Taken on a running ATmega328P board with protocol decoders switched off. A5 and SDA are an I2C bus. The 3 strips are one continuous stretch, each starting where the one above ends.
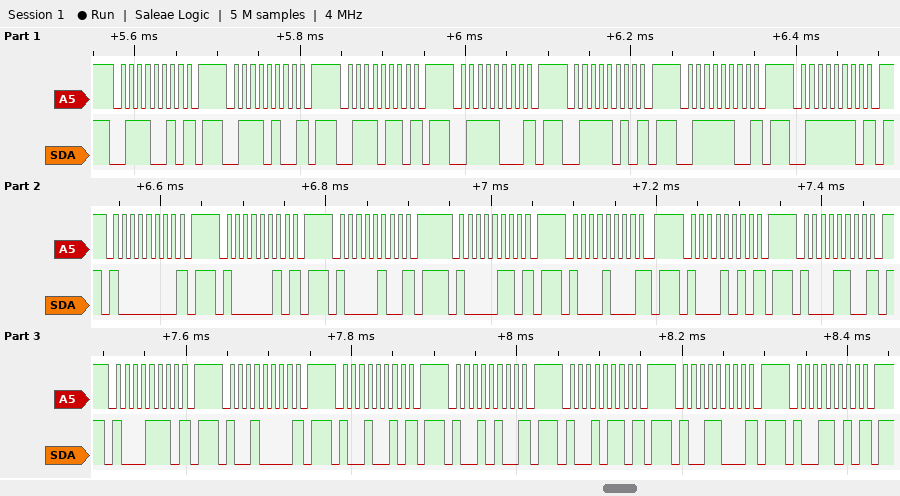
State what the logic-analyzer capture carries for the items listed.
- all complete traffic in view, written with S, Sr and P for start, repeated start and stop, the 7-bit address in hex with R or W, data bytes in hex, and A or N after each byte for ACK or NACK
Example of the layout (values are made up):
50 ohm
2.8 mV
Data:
S 39W N P S 3AW N P S 3BW N P S 3CW N P S 3DW N P S 3EW N P S 3FW N P S 40W N P S 41W N P S 42W N P S 43W N P S 44W N P S 45W N P S 46W N P S 47W N P S 48W N P S 49W N P S 4AW N P S 4BW N P S 4CW N P S 4DW N P
